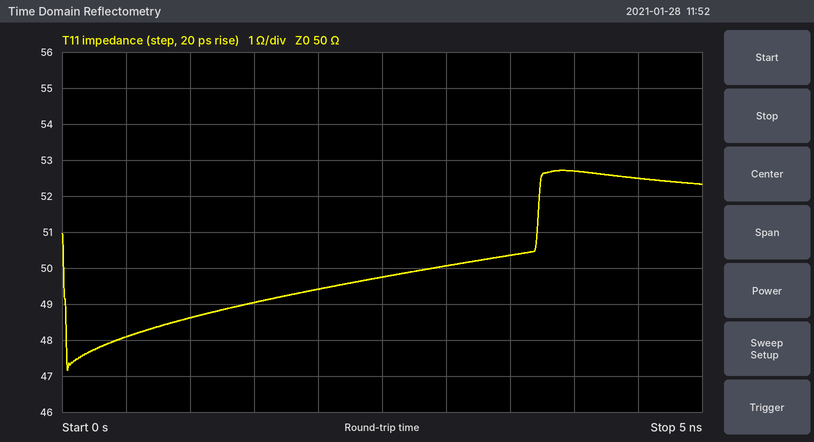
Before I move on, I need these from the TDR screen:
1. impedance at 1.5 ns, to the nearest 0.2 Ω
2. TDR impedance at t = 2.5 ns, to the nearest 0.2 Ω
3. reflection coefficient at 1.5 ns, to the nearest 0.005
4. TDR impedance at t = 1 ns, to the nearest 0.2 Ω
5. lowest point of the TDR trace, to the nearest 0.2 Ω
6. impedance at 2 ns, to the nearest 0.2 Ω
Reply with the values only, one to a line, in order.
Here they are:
49.0 Ω
49.8 Ω
-0.010
48.6 Ω
47.2 Ω
49.4 Ω
